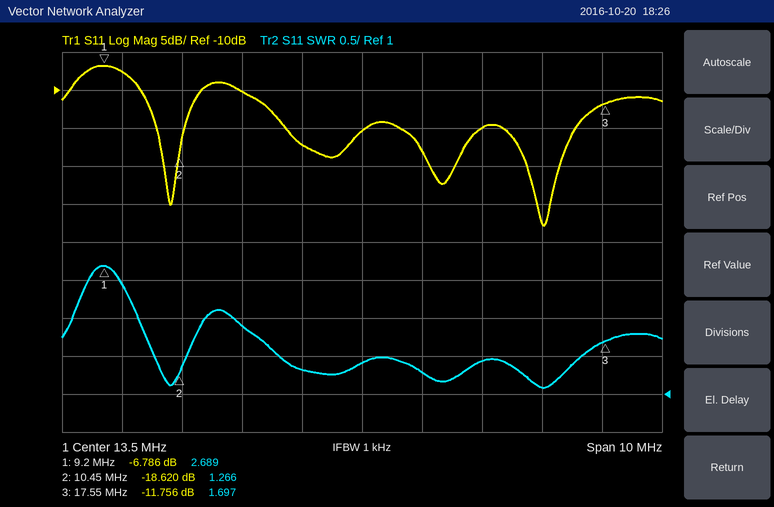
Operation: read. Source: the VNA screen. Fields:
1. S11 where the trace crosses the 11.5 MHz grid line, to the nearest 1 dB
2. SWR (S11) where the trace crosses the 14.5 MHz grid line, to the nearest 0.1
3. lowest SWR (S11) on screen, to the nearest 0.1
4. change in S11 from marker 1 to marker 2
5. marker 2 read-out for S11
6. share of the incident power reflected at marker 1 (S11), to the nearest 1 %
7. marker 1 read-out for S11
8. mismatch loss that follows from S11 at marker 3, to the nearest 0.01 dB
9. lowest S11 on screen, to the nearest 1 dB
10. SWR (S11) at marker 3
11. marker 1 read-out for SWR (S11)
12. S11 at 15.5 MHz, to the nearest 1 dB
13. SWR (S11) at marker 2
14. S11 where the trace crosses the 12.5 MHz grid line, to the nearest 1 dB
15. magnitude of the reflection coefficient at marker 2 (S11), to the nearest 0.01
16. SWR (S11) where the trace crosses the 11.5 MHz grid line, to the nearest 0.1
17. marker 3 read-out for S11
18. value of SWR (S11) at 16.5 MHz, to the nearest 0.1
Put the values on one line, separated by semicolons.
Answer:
-10 dB; 1.3; 1.1; -11.834 dB; -18.620 dB; 21 %; -6.786 dB; 0.30 dB; -28 dB; 1.697; 2.689; -15 dB; 1.266; -17 dB; 0.12; 1.9; -11.756 dB; 1.1
